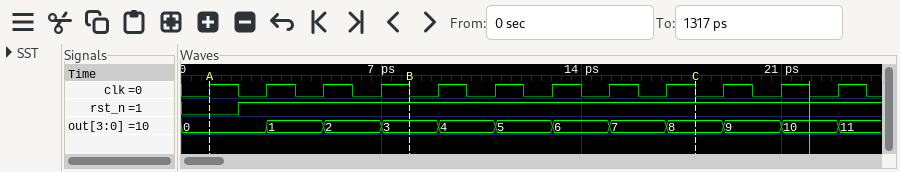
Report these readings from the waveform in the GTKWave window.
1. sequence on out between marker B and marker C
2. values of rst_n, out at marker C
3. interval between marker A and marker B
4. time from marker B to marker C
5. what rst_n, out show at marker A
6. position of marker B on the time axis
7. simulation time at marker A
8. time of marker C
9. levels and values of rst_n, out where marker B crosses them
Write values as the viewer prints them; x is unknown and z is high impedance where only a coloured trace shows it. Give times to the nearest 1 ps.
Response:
3, 4, 5, 6, 7, 8
rst_n=1, out=8
7 ps
10 ps
rst_n=0, out=0
8 ps
1 ps
18 ps
rst_n=1, out=3
